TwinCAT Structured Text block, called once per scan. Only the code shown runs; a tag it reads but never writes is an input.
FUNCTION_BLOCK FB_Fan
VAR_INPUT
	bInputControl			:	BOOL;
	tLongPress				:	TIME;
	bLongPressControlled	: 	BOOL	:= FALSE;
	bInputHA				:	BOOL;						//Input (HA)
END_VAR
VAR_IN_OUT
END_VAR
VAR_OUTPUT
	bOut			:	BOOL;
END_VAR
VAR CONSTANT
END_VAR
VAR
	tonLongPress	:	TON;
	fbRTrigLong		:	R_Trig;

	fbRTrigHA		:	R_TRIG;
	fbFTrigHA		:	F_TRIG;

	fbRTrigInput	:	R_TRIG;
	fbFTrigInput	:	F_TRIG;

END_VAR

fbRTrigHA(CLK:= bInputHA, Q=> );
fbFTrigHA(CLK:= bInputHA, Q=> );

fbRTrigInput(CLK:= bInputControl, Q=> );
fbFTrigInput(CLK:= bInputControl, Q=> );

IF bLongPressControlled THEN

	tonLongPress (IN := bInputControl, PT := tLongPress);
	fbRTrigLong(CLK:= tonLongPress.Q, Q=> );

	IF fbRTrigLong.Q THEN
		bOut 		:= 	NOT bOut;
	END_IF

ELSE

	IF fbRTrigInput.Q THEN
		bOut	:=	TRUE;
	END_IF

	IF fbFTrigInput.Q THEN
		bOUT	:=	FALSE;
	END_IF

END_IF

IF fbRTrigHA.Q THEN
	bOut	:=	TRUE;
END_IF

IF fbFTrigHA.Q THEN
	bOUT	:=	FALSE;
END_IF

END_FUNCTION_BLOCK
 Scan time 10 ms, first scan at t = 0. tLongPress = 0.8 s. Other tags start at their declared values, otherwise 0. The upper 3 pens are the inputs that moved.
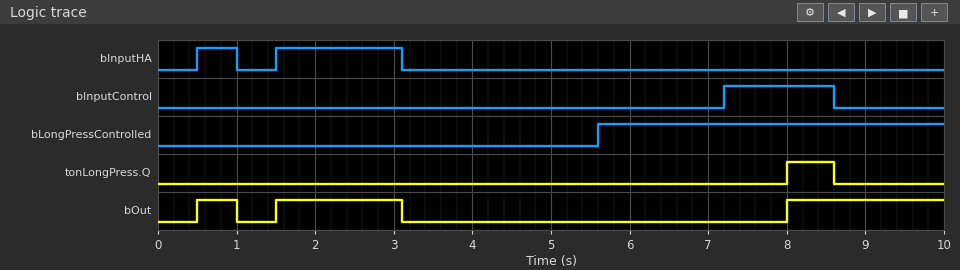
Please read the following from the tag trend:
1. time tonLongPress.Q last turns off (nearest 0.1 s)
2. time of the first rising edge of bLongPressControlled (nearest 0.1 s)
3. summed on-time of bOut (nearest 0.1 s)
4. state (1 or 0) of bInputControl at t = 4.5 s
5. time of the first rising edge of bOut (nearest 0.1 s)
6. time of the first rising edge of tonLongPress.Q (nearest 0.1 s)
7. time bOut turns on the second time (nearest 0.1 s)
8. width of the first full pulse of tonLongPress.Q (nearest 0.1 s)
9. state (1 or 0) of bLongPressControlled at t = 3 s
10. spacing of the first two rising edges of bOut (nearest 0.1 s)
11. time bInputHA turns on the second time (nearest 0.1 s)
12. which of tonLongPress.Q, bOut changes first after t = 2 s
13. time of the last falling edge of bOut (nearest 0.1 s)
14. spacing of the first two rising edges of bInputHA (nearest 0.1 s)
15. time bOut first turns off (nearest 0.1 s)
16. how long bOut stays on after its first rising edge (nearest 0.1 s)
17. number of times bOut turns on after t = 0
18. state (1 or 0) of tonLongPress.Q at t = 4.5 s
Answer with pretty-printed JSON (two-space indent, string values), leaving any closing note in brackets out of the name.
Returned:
{
  "time tonLongPress.Q last turns off": "8.6 s",
  "time of the first rising edge of bLongPressControlled": "5.6 s",
  "summed on-time of bOut": "4.1 s",
  "state (1 or 0) of bInputControl at t = 4.5 s": "0",
  "time of the first rising edge of bOut": "0.5 s",
  "time of the first rising edge of tonLongPress.Q": "8.0 s",
  "time bOut turns on the second time": "1.5 s",
  "width of the first full pulse of tonLongPress.Q": "0.6 s",
  "state (1 or 0) of bLongPressControlled at t = 3 s": "0",
  "spacing of the first two rising edges of bOut": "1.0 s",
  "time bInputHA turns on the second time": "1.5 s",
  "which of tonLongPress.Q, bOut changes first after t = 2 s": "bOut",
  "time of the last falling edge of bOut": "3.1 s",
  "spacing of the first two rising edges of bInputHA": "1.0 s",
  "time bOut first turns off": "1.0 s",
  "how long bOut stays on after its first rising edge": "0.5 s",
  "number of times bOut turns on after t = 0": "3",
  "state (1 or 0) of tonLongPress.Q at t = 4.5 s": "0"
}
